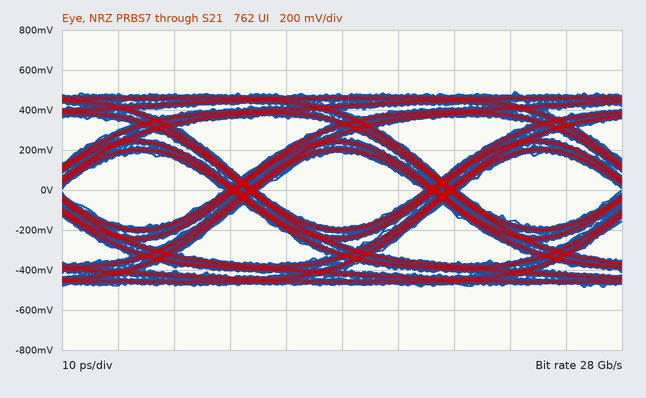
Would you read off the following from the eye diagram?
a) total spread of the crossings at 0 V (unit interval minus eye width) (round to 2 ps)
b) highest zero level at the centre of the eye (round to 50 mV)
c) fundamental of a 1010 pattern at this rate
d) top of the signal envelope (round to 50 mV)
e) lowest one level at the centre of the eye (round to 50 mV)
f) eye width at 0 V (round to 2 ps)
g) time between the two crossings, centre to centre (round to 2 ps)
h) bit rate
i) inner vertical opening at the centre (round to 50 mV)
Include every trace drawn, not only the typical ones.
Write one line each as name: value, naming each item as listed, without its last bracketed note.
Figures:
total spread of the crossings at 0 V (unit interval minus eye width): 6 ps
highest zero level at the centre of the eye: -200 mV
fundamental of a 1010 pattern at this rate: 14 GHz
top of the signal envelope: 500 mV
lowest one level at the centre of the eye: 200 mV
eye width at 0 V: 30 ps
time between the two crossings, centre to centre: 36 ps
bit rate: 28 Gb/s
inner vertical opening at the centre: 400 mV
